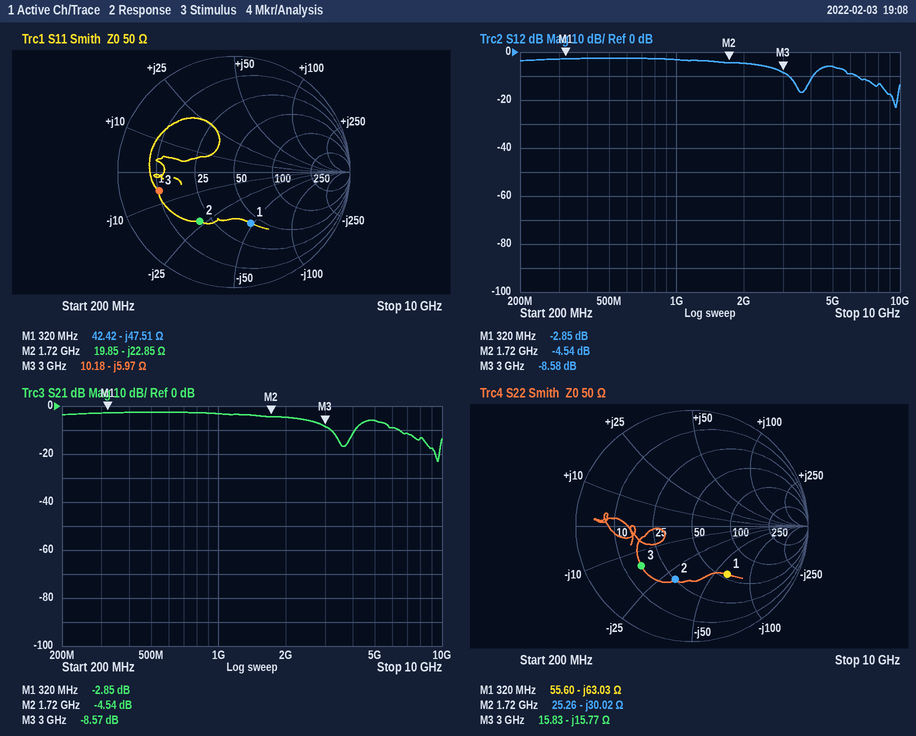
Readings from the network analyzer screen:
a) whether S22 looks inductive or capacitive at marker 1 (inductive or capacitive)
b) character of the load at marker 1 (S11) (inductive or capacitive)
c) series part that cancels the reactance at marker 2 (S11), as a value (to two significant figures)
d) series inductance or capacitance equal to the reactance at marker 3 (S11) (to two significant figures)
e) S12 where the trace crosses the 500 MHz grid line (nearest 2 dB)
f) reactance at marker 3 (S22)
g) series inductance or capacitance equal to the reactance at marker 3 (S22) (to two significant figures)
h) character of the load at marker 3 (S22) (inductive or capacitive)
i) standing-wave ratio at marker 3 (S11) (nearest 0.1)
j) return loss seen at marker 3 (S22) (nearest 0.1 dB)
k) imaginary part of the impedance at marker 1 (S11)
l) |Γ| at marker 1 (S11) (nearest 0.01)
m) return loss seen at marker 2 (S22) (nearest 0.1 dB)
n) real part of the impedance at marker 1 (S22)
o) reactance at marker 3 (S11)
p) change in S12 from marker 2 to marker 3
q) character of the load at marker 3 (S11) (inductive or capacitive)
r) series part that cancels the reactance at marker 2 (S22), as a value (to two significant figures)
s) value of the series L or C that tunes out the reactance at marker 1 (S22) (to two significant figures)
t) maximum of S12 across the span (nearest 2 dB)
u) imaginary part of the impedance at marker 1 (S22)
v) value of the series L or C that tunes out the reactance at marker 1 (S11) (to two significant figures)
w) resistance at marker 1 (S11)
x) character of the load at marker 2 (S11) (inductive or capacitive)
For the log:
capacitive
capacitive
2.1 nH
8.9 pF
-2 dB
-15.77 Ω
3.4 pF
capacitive
5.0
5.1 dB
-47.51 Ω
0.46
6.4 dB
55.60 Ω
-5.97 Ω
-4.04 dB
capacitive
2.8 nH
31 nH
-2 dB
-63.03 Ω
24 nH
42.42 Ω
capacitive
